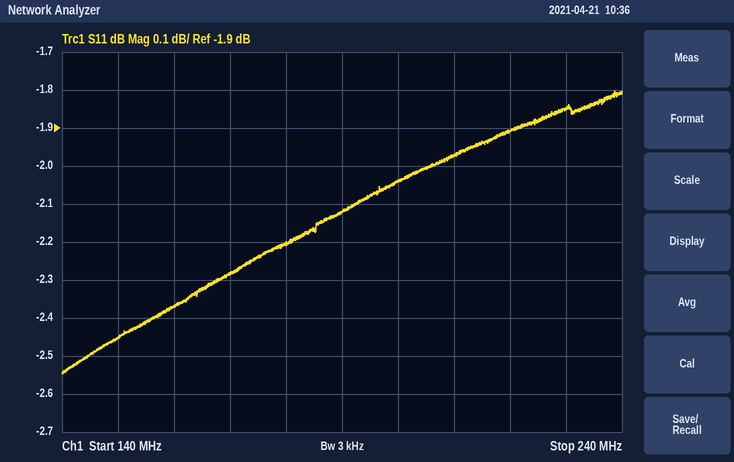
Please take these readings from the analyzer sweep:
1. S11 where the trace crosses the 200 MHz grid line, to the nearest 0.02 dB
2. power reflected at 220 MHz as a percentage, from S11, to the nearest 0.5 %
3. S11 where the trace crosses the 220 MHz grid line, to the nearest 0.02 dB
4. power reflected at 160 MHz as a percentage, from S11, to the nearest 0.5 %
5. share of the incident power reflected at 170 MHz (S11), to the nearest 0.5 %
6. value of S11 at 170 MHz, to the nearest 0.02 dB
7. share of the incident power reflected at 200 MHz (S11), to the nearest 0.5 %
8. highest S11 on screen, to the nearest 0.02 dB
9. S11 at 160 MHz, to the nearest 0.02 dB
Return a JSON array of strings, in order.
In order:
["-2.04 dB", "64.5 %", "-1.90 dB", "58.0 %", "59.0 %", "-2.28 dB", "62.5 %", "-1.80 dB", "-2.36 dB"]
